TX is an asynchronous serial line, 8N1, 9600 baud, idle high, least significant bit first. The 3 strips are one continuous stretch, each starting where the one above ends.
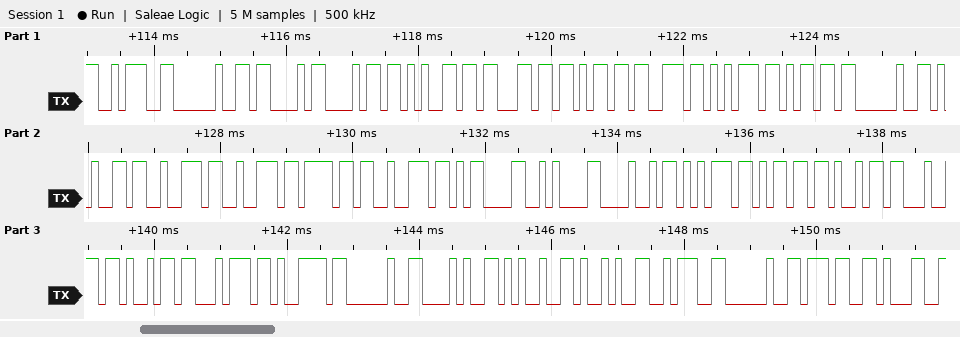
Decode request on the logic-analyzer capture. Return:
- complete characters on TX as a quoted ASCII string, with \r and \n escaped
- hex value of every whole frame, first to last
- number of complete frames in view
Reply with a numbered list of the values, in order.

1. ": Checksum error\r\nHumidity (%): 71"
2. 3A 20 43 68 65 63 6B 73 75 6D 20 65 72 72 6F 72 0D 0A 48 75 6D 69 64 69 74 79 20 28 25 29 3A 20 37 31
3. 34
